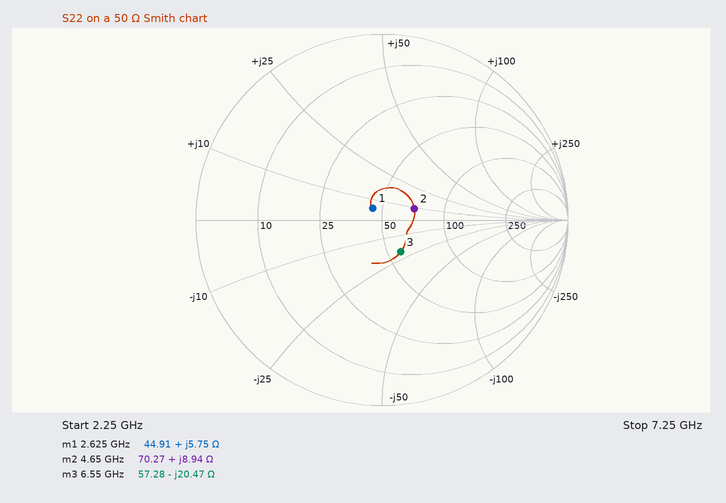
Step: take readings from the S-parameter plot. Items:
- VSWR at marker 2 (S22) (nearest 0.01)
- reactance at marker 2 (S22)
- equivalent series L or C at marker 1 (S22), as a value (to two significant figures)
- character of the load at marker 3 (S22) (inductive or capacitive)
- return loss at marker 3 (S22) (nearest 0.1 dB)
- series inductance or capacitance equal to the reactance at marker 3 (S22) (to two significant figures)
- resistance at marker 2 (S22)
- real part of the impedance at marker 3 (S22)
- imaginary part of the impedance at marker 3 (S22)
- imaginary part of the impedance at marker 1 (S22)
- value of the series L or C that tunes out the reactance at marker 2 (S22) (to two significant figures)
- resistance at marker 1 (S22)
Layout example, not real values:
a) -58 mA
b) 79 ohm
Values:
a) 1.45
b) +8.94 Ω
c) 350 pH
d) capacitive
e) 14.0 dB
f) 1.2 pF
g) 70.27 Ω
h) 57.28 Ω
i) -20.47 Ω
j) +5.75 Ω
k) 3.8 pF
l) 44.91 Ω
